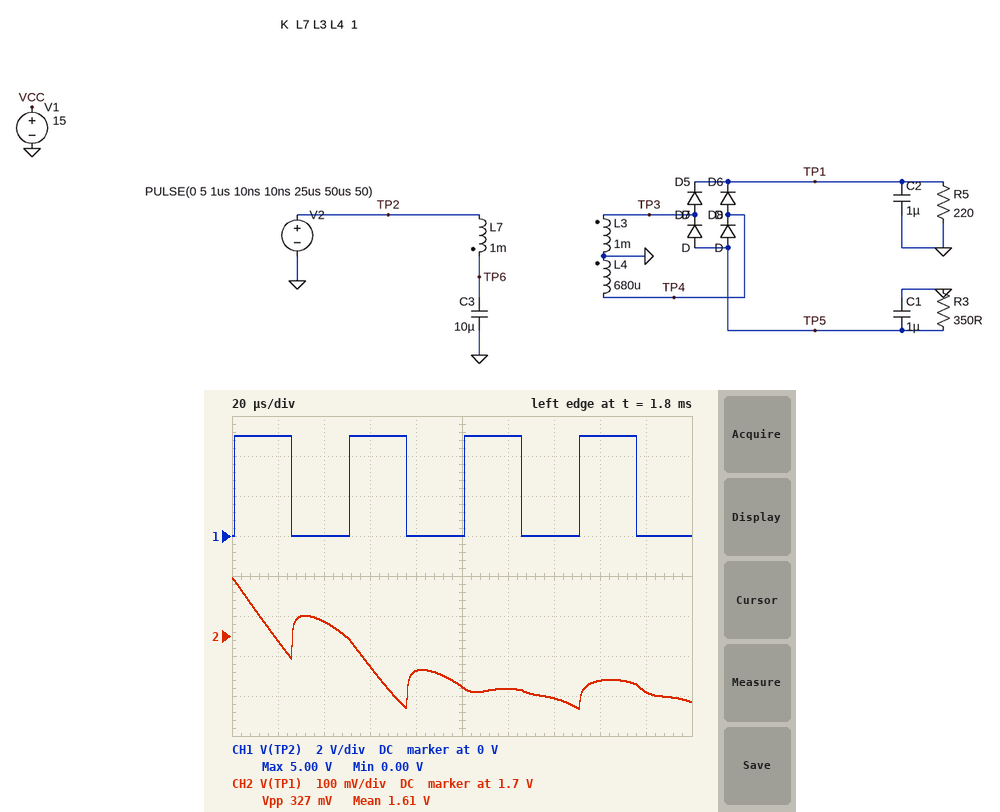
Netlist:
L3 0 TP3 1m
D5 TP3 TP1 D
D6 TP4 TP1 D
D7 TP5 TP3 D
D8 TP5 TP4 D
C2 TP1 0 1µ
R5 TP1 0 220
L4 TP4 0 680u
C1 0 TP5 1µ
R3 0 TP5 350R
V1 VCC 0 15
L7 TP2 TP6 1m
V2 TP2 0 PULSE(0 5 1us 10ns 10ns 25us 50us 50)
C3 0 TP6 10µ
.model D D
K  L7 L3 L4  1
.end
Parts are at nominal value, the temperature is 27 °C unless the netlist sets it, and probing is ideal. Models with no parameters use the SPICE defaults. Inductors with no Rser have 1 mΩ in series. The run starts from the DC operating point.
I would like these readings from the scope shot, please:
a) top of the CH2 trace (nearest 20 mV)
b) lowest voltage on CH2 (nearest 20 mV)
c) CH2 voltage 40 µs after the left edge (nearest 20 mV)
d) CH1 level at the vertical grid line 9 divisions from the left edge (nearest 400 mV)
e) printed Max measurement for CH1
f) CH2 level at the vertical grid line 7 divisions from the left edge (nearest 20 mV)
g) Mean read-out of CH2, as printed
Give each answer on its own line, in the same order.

1.84 V
1.52 V
1.74 V
0 V
5.00 V
1.54 V
1.61 V
